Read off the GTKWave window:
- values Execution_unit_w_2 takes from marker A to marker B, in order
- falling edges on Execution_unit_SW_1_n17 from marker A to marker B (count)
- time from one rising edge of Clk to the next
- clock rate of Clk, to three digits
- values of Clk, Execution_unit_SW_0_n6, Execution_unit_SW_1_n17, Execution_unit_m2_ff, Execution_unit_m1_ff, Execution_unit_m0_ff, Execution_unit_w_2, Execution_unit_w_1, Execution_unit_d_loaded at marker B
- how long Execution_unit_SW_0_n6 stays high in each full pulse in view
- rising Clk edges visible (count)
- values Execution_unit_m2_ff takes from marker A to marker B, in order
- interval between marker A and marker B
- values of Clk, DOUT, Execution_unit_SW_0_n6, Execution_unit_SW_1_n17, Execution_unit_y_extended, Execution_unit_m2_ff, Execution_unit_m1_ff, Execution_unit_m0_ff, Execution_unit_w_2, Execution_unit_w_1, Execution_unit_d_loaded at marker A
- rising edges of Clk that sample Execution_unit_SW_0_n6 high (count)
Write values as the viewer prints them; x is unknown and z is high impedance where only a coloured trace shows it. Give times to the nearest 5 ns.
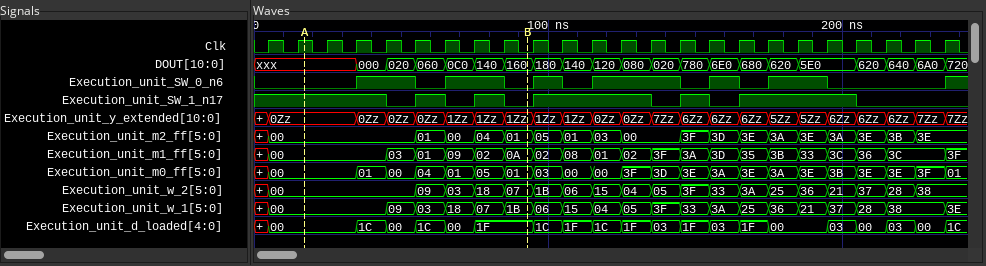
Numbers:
00, 09, 03, 18, 07
3
10 ns
100 MHz
Clk=0, Execution_unit_SW_0_n6=0, Execution_unit_SW_1_n17=0, Execution_unit_m2_ff=01, Execution_unit_m1_ff=0A, Execution_unit_m0_ff=01, Execution_unit_w_2=07, Execution_unit_w_1=1B, Execution_unit_d_loaded=1F
20 ns, 20 ns, 10 ns, 30 ns, 10 ns, 20 ns
24
00, 01, 00, 04, 01
75 ns
Clk=1, DOUT=xxx, Execution_unit_SW_0_n6=0, Execution_unit_SW_1_n17=1, Execution_unit_y_extended=0Zz, Execution_unit_m2_ff=00, Execution_unit_m1_ff=00, Execution_unit_m0_ff=00, Execution_unit_w_2=00, Execution_unit_w_1=00, Execution_unit_d_loaded=00
11
